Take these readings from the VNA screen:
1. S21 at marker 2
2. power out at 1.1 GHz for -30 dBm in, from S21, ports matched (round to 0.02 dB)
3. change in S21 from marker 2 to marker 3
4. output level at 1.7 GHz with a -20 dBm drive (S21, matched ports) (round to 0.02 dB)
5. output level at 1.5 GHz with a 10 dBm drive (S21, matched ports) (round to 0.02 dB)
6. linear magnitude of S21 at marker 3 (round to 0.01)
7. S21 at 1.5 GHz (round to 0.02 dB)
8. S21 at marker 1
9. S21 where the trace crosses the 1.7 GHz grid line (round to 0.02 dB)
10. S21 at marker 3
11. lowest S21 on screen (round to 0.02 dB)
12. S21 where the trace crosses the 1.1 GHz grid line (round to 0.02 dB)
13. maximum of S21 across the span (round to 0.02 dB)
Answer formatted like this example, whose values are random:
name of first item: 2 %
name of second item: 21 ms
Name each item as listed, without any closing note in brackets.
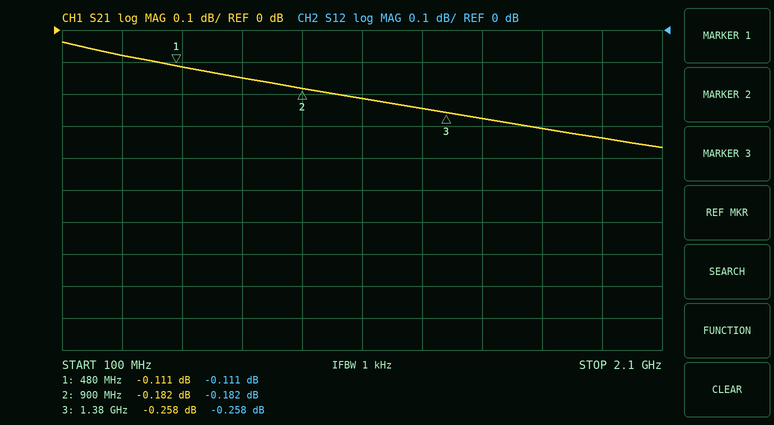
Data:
S21 at marker 2: -0.182 dB
power out at 1.1 GHz for -30 dBm in, from S21, ports matched: -30.22 dBm
change in S21 from marker 2 to marker 3: -0.076 dB
output level at 1.7 GHz with a -20 dBm drive (S21, matched ports): -20.30 dBm
output level at 1.5 GHz with a 10 dBm drive (S21, matched ports): 9.72 dBm
linear magnitude of S21 at marker 3: 0.97
S21 at 1.5 GHz: -0.28 dB
S21 at marker 1: -0.111 dB
S21 where the trace crosses the 1.7 GHz grid line: -0.30 dB
S21 at marker 3: -0.258 dB
lowest S21 on screen: -0.36 dB
S21 where the trace crosses the 1.1 GHz grid line: -0.22 dB
maximum of S21 across the span: -0.04 dB
